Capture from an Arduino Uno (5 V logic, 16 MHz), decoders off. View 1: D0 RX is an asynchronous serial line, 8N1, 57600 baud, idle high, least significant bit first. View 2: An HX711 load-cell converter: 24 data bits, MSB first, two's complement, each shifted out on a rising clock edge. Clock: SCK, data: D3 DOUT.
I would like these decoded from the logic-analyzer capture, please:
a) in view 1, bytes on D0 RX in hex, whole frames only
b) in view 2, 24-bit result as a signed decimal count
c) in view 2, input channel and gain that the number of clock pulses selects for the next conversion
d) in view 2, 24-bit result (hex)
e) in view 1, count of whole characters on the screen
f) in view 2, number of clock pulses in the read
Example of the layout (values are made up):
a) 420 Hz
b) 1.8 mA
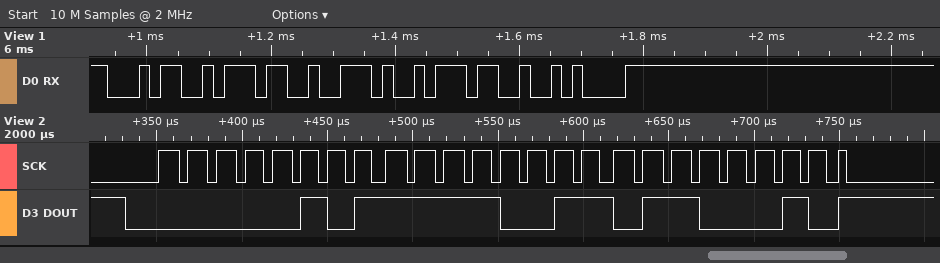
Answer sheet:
a) 0x34 0x37 0x2E 0x37 0x0A
b) 389986
c) channel A, gain 128
d) 0x05F362
e) 5
f) 25
